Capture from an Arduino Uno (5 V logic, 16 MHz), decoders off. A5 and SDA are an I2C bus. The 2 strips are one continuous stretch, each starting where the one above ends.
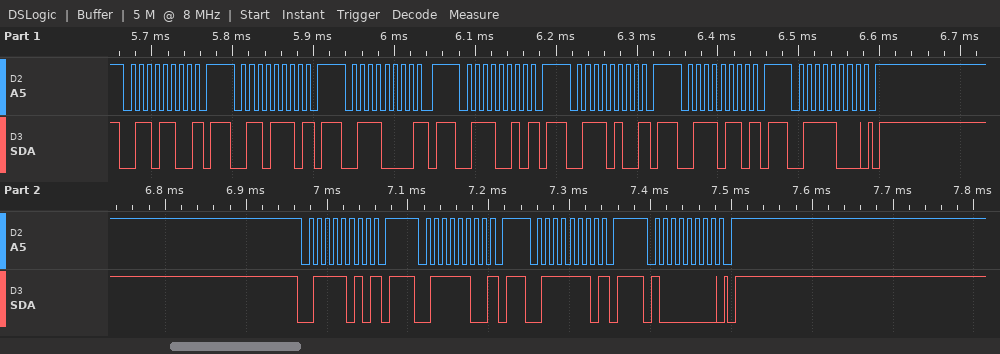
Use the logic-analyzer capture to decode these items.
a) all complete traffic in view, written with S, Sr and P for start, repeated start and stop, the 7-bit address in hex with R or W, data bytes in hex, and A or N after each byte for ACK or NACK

S 36W N P S 37W N P S 38W N P S 39W N P S 3AW N P S 3BW N P S 3CW A P S 3DW N P S 3EW N P S 3FW N P S 40W A P
